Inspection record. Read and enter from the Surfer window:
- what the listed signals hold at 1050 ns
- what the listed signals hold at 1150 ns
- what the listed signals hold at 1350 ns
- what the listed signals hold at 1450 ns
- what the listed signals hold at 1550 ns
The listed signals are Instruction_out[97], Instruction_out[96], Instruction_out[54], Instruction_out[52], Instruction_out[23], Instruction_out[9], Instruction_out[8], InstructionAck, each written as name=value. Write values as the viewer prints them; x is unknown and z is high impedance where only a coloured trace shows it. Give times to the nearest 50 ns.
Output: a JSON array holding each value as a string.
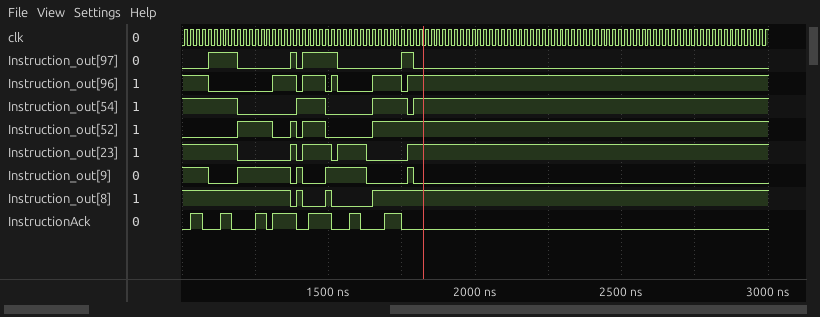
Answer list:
["Instruction_out[97]=0, Instruction_out[96]=1, Instruction_out[54]=1, Instruction_out[52]=0, Instruction_out[23]=1, Instruction_out[9]=1, Instruction_out[8]=1, InstructionAck=1", "Instruction_out[97]=1, Instruction_out[96]=0, Instruction_out[54]=1, Instruction_out[52]=0, Instruction_out[23]=1, Instruction_out[9]=0, Instruction_out[8]=1, InstructionAck=1", "Instruction_out[97]=0, Instruction_out[96]=1, Instruction_out[54]=0, Instruction_out[52]=0, Instruction_out[23]=0, Instruction_out[9]=1, Instruction_out[8]=1, InstructionAck=1", "Instruction_out[97]=1, Instruction_out[96]=1, Instruction_out[54]=1, Instruction_out[52]=1, Instruction_out[23]=1, Instruction_out[9]=0, Instruction_out[8]=0, InstructionAck=1", "Instruction_out[97]=0, Instruction_out[96]=0, Instruction_out[54]=0, Instruction_out[52]=0, Instruction_out[23]=1, Instruction_out[9]=1, Instruction_out[8]=0, InstructionAck=0"]
